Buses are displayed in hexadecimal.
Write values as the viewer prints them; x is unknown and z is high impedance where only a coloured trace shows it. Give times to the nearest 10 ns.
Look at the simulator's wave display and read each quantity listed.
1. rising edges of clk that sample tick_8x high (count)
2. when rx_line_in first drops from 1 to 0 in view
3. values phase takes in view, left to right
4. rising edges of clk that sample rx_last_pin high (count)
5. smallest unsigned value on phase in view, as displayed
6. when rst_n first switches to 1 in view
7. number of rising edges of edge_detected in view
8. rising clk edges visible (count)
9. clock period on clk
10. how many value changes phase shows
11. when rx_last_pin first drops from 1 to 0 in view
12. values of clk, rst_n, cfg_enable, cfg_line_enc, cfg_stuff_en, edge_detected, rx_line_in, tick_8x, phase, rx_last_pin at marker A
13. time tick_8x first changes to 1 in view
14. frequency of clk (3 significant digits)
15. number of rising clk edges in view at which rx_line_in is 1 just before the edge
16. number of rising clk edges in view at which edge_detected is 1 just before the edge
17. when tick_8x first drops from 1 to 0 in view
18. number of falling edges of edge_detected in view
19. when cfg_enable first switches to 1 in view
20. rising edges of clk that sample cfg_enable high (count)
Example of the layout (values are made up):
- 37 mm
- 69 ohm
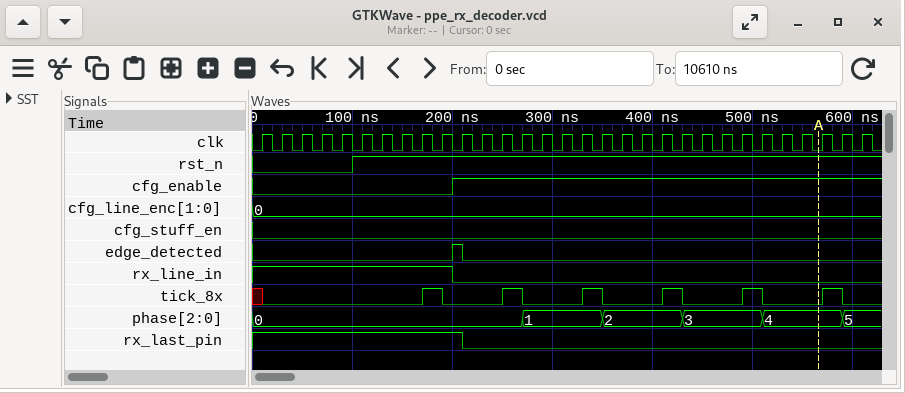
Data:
- 6
- 200 ns
- 0, 1, 2, 3, 4, 5
- 11
- 0
- 100 ns
- 1
- 31
- 20 ns
- 5
- 210 ns
- clk=0, rst_n=1, cfg_enable=1, cfg_line_enc=0, cfg_stuff_en=0, edge_detected=0, rx_line_in=0, tick_8x=0, phase=4, rx_last_pin=0
- 170 ns
- 50.0 MHz
- 10
- 1
- 190 ns
- 1
- 200 ns
- 21
